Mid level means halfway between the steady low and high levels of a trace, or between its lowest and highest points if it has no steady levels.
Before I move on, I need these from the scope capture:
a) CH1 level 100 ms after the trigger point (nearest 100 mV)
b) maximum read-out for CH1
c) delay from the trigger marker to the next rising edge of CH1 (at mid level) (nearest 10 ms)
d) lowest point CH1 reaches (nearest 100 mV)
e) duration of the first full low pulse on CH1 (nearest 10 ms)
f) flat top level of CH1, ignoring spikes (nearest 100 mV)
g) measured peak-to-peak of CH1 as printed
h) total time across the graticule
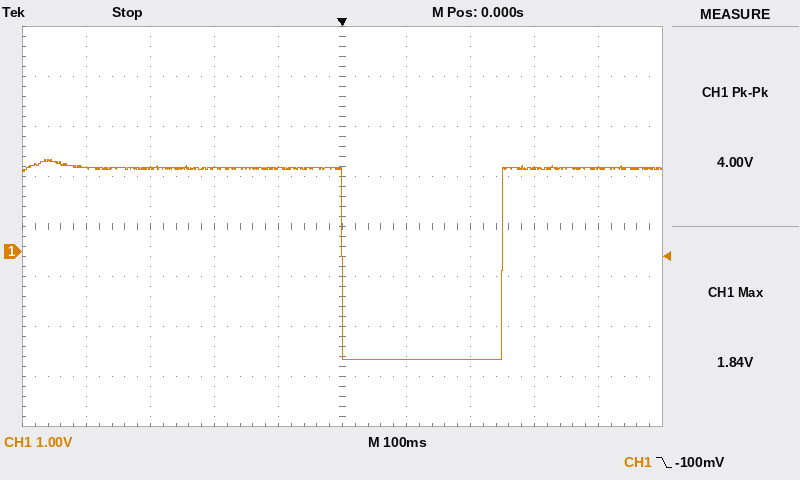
-2.2 V
1.84 V
250 ms
-2.2 V
250 ms
1.7 V
4.00 V
1 s
